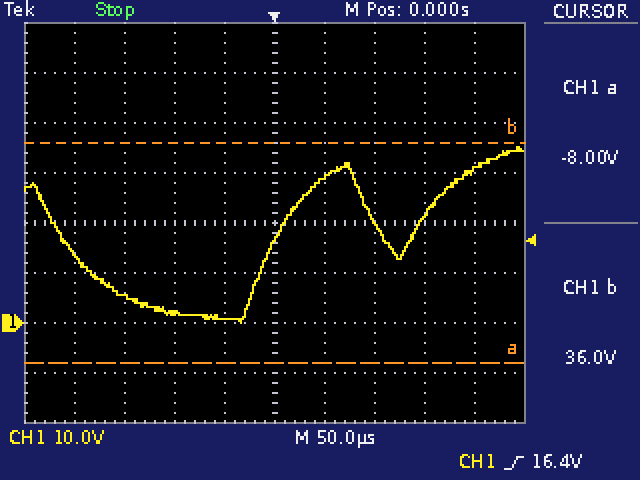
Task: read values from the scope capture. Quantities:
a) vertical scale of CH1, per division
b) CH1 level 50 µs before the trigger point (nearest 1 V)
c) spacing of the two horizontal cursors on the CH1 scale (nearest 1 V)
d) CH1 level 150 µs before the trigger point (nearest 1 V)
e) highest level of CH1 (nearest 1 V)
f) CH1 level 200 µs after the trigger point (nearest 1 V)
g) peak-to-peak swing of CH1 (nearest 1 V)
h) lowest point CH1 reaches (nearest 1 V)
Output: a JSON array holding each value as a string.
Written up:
["10 V", "1 V", "44 V", "5 V", "35 V", "30 V", "35 V", "0 V"]
